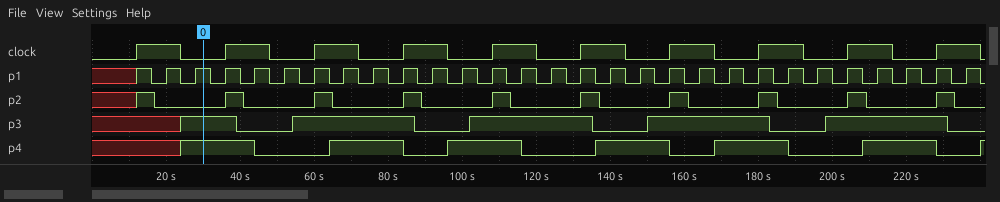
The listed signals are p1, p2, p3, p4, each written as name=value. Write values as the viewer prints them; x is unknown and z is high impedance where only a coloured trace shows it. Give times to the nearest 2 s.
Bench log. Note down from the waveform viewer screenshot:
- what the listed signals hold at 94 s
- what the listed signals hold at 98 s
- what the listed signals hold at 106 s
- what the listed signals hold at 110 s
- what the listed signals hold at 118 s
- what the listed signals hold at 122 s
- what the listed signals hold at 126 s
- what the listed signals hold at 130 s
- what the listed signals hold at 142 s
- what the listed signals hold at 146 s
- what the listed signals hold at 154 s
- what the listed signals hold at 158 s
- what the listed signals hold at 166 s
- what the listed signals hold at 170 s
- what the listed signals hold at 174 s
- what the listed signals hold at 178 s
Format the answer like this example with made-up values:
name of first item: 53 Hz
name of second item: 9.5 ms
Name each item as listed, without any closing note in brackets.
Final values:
what the listed signals hold at 94 s: p1=1, p2=0, p3=0, p4=0
what the listed signals hold at 98 s: p1=0, p2=0, p3=0, p4=1
what the listed signals hold at 106 s: p1=0, p2=0, p3=1, p4=1
what the listed signals hold at 110 s: p1=1, p2=1, p3=1, p4=1
what the listed signals hold at 118 s: p1=1, p2=0, p3=1, p4=0
what the listed signals hold at 122 s: p1=0, p2=0, p3=1, p4=0
what the listed signals hold at 126 s: p1=1, p2=0, p3=1, p4=0
what the listed signals hold at 130 s: p1=0, p2=0, p3=1, p4=0
what the listed signals hold at 142 s: p1=1, p2=0, p3=0, p4=1
what the listed signals hold at 146 s: p1=0, p2=0, p3=0, p4=1
what the listed signals hold at 154 s: p1=0, p2=0, p3=1, p4=1
what the listed signals hold at 158 s: p1=1, p2=1, p3=1, p4=0
what the listed signals hold at 166 s: p1=1, p2=0, p3=1, p4=0
what the listed signals hold at 170 s: p1=0, p2=0, p3=1, p4=1
what the listed signals hold at 174 s: p1=1, p2=0, p3=1, p4=1
what the listed signals hold at 178 s: p1=0, p2=0, p3=1, p4=1
